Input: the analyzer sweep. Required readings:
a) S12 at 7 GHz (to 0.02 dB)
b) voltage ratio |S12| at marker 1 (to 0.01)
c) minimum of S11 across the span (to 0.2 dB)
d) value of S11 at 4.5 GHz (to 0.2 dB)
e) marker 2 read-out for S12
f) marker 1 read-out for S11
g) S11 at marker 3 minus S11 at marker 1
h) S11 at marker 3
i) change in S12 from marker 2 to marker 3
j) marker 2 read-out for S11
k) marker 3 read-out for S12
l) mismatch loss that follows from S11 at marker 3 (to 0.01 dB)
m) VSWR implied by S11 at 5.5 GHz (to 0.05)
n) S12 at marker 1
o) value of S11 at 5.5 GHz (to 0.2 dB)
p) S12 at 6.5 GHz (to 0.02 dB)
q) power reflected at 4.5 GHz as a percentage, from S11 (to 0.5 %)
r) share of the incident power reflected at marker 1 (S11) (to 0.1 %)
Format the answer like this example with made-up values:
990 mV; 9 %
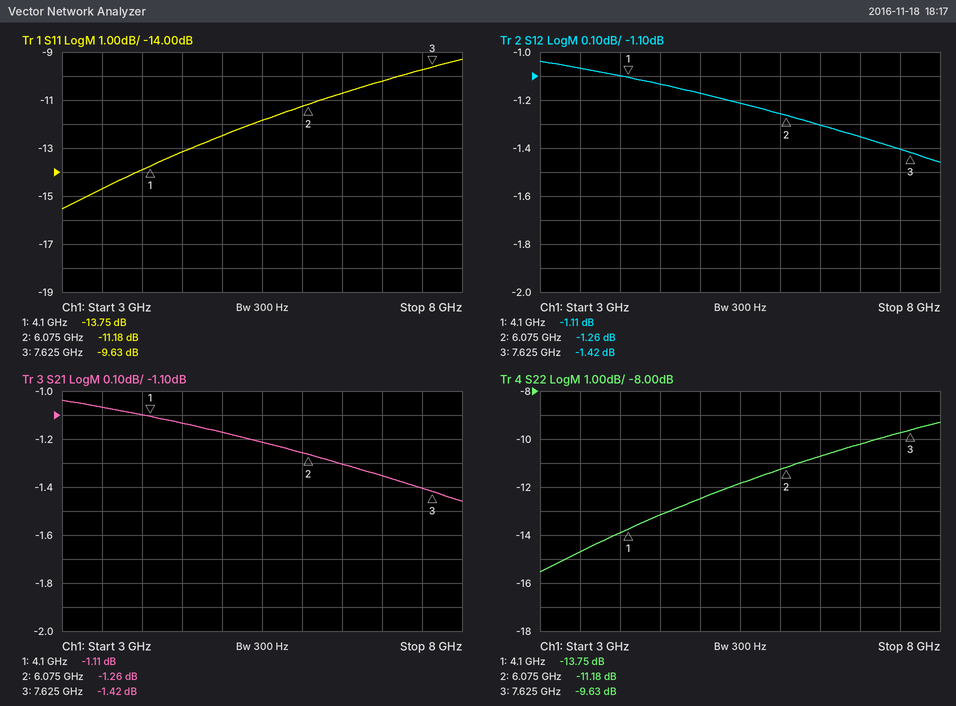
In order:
-1.36 dB; 0.88; -15.6 dB; -13.2 dB; -1.26 dB; -13.75 dB; 4.12 dB; -9.63 dB; -0.16 dB; -11.18 dB; -1.42 dB; 0.50 dB; 1.70; -1.11 dB; -11.8 dB; -1.30 dB; 5.0 %; 4.2 %
